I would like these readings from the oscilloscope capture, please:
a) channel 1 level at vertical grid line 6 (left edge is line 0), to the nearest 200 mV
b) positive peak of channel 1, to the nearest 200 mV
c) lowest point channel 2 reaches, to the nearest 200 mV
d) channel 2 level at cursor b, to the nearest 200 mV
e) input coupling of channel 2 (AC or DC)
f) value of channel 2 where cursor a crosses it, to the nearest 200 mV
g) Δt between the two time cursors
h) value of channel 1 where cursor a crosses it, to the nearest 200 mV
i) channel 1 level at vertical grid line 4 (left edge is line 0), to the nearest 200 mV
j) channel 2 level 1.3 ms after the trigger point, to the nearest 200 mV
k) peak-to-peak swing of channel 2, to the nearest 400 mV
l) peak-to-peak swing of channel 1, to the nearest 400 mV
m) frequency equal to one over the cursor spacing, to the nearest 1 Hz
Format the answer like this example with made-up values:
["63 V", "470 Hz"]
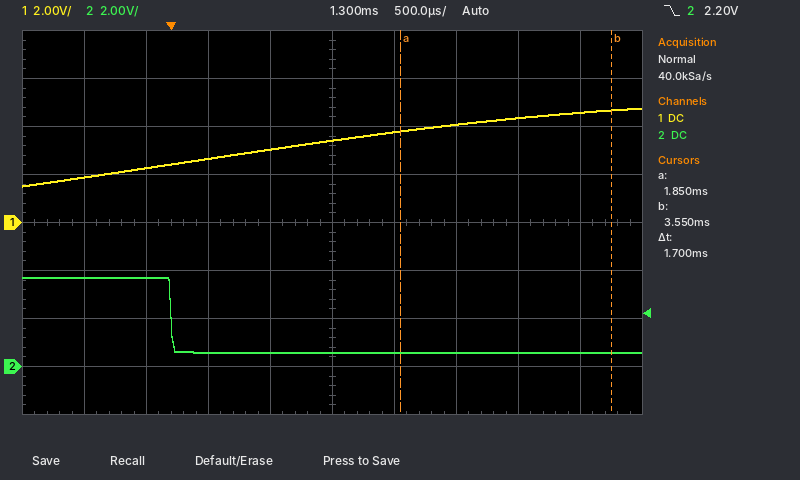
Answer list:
["3.8 V", "4.8 V", "600 mV", "600 mV", "DC", "600 mV", "1.7 ms", "3.8 V", "3.0 V", "600 mV", "3.2 V", "3.2 V", "588 Hz"]
